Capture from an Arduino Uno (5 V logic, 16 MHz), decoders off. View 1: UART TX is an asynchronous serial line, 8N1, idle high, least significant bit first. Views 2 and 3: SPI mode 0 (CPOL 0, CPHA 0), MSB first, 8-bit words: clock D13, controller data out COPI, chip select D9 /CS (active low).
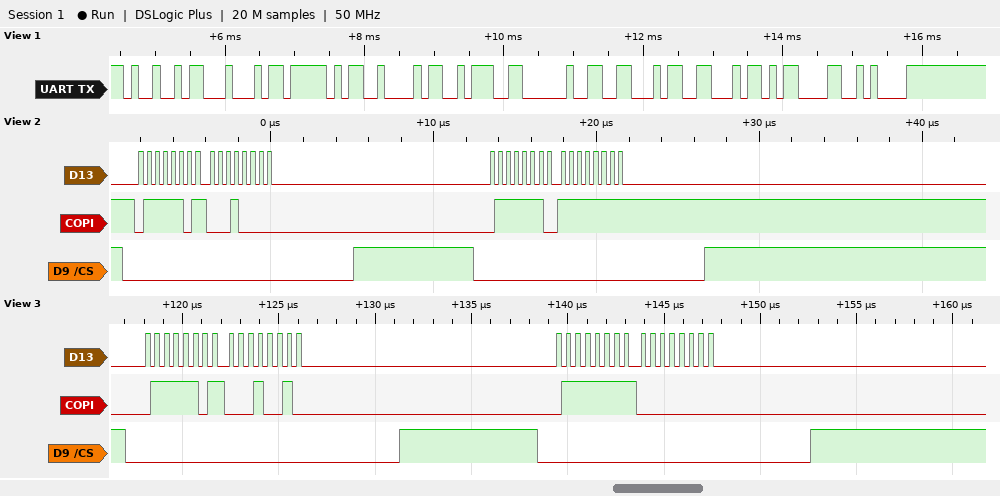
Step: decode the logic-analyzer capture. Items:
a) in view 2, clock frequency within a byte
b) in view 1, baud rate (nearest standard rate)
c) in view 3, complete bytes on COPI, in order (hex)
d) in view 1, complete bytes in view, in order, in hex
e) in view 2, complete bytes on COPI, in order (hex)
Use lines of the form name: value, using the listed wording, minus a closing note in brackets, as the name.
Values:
in view 2, clock frequency within a byte: 2 MHz
in view 1, baud rate: 9600 baud
in view 3, complete bytes on COPI, in order: 7D 12 7F 00
in view 1, complete bytes in view, in order, in hex: 49 44 5F 42 3A 20 46 46 0D 0A
in view 2, complete bytes on COPI, in order: 7D 10 7E FF
